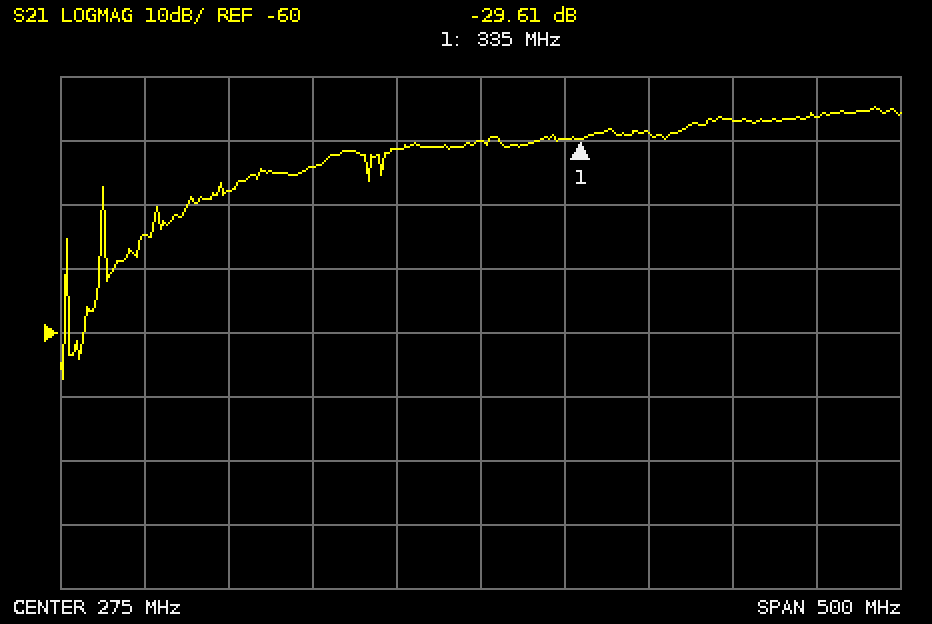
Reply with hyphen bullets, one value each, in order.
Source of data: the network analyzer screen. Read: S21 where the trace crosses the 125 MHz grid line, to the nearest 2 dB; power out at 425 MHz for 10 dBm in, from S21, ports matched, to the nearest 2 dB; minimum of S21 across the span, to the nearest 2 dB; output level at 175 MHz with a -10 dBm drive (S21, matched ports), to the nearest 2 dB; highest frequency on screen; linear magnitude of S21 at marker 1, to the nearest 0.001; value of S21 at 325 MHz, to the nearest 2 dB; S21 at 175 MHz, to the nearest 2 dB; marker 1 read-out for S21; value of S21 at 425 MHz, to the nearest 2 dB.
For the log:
- -38 dB
- -16 dBm
- -68 dB
- -44 dBm
- 525 MHz
- 0.033
- -30 dB
- -34 dB
- -29.61 dB
- -26 dB
